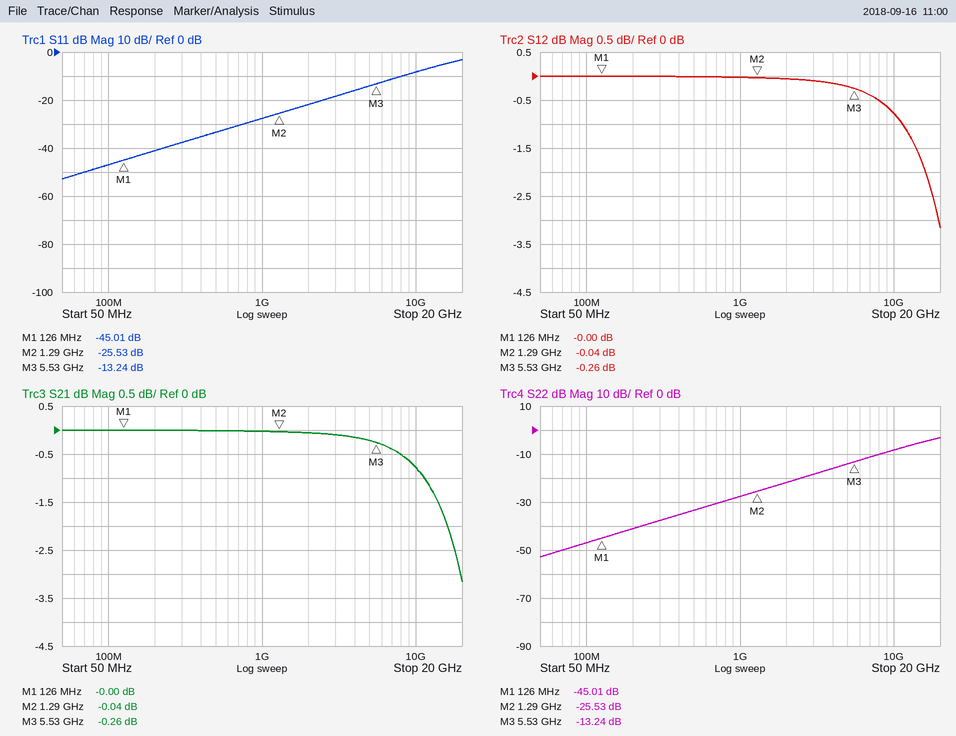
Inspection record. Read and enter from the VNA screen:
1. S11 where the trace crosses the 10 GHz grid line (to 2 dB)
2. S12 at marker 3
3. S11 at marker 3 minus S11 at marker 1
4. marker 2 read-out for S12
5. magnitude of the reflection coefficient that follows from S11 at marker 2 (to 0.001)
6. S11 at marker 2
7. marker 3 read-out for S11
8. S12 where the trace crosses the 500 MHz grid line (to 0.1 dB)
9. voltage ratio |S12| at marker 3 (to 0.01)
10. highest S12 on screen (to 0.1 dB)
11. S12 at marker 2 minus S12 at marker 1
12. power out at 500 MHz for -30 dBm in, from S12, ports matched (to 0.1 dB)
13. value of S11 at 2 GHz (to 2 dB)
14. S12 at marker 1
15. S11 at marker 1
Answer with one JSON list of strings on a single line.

["-8 dB", "-0.26 dB", "31.77 dB", "-0.04 dB", "0.053", "-25.53 dB", "-13.24 dB", "0.0 dB", "0.97", "0.0 dB", "-0.04 dB", "-30.0 dBm", "-22 dB", "-0.00 dB", "-45.01 dB"]
